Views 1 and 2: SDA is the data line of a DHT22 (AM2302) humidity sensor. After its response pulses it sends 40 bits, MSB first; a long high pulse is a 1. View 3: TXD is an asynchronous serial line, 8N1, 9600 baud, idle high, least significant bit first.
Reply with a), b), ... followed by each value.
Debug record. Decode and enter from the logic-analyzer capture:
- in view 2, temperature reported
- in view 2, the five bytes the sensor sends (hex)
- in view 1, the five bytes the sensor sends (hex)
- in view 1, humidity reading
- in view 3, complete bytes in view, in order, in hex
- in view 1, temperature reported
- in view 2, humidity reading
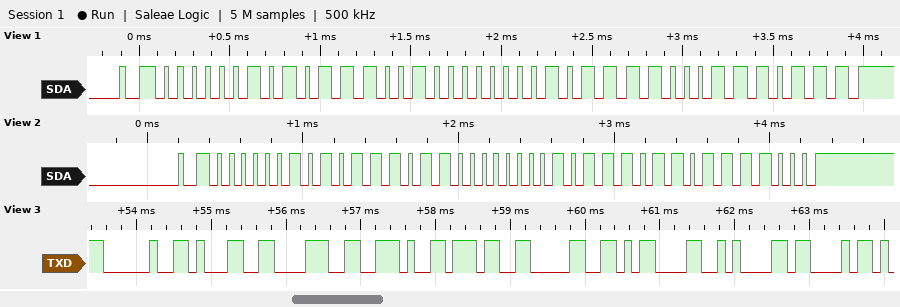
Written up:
a) 18.7 °C
b) 02 BB 00 BB 78
c) 02 B9 00 BC 77
d) 69.7 %
e) 20 31 38 2E 37 30 0D 0A 43
f) 18.8 °C
g) 69.9 %
